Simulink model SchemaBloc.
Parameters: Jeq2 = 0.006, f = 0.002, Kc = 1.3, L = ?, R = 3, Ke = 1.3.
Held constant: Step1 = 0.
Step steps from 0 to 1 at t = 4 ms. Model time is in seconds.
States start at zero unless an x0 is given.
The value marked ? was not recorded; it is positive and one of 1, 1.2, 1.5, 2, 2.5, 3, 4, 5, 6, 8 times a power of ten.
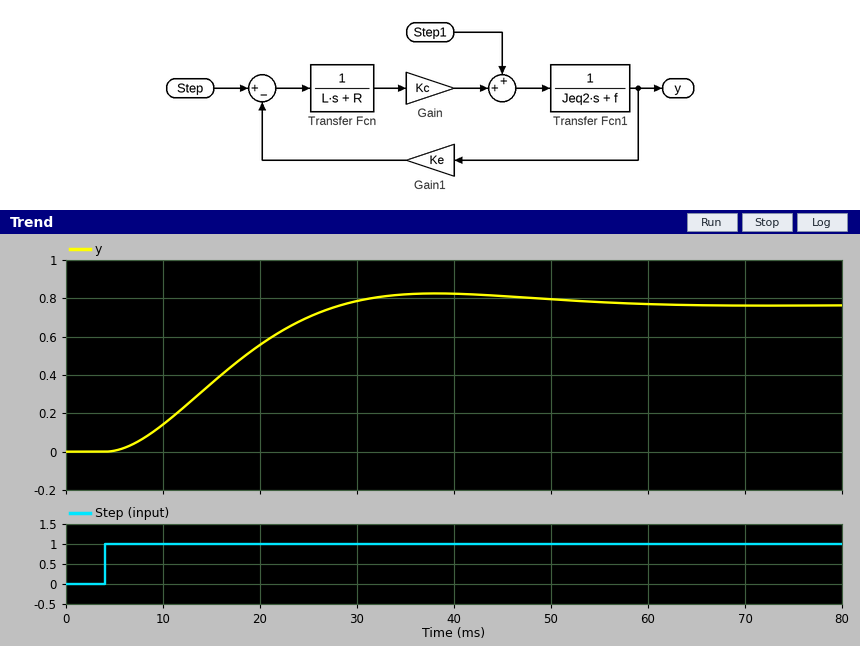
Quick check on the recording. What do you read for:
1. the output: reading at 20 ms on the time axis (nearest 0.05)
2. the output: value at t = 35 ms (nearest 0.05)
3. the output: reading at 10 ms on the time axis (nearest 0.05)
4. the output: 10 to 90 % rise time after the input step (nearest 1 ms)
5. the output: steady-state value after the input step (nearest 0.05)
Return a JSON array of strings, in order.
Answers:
["0.55", "0.80", "0.15", "16 ms", "0.75"]
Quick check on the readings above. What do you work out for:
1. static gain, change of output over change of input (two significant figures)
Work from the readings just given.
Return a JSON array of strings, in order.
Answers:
["0.75"]
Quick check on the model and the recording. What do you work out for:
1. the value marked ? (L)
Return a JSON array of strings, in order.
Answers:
["0.02"]
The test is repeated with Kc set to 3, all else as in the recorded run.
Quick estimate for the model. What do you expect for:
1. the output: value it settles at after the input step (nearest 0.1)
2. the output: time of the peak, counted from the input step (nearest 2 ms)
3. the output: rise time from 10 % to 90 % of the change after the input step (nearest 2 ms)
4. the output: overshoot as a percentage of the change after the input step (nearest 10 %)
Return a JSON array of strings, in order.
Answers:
["0.8", "20 ms", "8 ms", "20 %"]
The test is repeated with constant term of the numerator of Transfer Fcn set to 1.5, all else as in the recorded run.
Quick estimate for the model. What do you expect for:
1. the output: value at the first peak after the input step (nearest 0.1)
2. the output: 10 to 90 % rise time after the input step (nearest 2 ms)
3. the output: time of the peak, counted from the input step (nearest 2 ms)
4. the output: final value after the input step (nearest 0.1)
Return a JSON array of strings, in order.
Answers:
["0.9", "12 ms", "26 ms", "0.8"]
